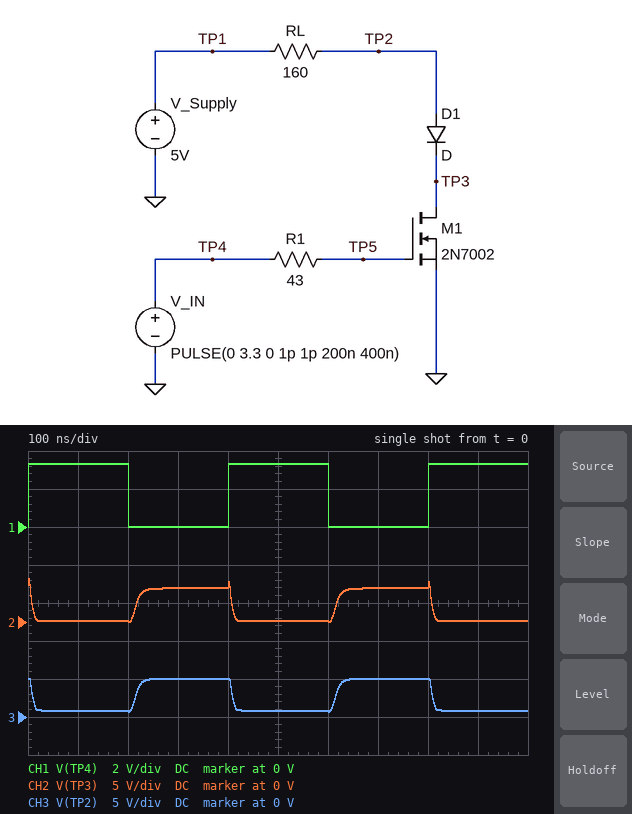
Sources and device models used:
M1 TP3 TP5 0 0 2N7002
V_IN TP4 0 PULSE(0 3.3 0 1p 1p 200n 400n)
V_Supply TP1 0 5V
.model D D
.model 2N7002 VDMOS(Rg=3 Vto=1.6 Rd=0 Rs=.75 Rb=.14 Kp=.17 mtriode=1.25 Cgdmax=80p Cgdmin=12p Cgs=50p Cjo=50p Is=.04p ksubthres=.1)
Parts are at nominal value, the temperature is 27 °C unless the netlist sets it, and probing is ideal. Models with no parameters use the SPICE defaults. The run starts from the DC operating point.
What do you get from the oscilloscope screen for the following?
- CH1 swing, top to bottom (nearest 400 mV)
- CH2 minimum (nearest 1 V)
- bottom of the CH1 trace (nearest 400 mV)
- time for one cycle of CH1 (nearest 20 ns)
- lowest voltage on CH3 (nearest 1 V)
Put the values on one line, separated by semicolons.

3.2 V; 0 V; 0 V; 400 ns; 1 V
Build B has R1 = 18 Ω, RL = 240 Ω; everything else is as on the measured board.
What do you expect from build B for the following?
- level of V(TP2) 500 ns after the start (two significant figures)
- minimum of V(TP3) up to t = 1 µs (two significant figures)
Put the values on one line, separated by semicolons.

790 mV; -540 mV
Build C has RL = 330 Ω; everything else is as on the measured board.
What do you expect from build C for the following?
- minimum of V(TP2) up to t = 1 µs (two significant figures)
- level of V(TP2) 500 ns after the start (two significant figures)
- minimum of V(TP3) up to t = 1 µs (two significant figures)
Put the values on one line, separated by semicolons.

470 mV; 770 mV; -250 mV
